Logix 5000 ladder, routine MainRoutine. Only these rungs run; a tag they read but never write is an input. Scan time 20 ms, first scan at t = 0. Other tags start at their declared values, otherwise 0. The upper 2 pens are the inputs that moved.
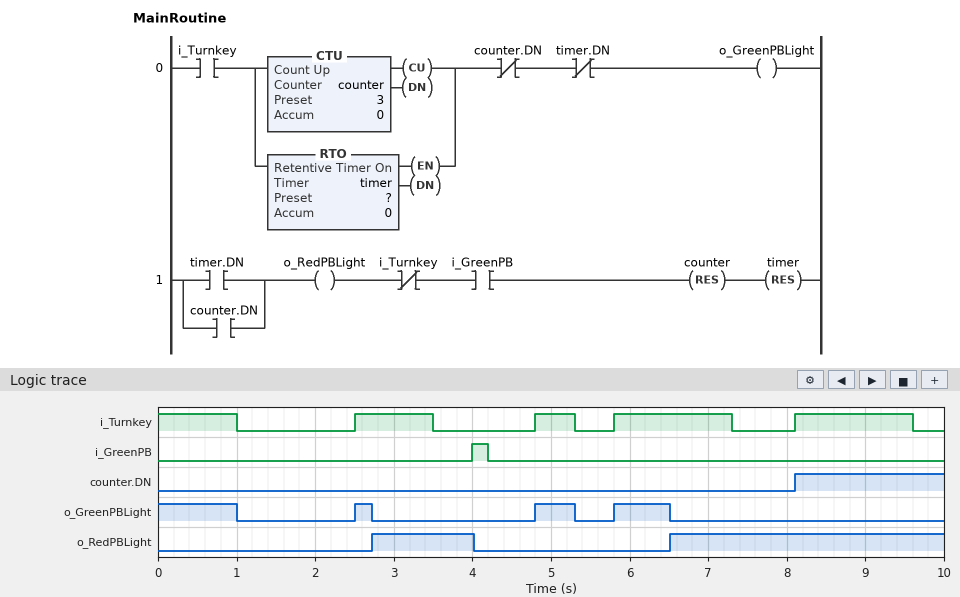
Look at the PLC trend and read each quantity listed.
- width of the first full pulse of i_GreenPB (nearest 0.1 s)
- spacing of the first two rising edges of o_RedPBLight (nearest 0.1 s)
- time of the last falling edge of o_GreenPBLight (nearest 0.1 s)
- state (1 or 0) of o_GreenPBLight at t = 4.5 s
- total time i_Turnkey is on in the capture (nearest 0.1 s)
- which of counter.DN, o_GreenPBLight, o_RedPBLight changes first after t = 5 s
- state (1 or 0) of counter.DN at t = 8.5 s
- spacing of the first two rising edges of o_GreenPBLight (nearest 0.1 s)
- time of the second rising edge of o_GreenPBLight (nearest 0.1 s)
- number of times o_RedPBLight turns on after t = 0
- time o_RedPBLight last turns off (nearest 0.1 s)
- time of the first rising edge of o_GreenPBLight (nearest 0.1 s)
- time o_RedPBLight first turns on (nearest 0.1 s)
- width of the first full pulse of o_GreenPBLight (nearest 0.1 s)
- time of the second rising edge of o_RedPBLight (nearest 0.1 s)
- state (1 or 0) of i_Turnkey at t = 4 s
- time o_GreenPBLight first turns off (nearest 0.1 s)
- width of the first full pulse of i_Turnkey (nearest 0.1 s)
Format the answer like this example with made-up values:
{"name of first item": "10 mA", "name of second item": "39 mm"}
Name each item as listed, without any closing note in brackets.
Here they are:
{"width of the first full pulse of i_GreenPB": "0.2 s", "spacing of the first two rising edges of o_RedPBLight": "3.8 s", "time of the last falling edge of o_GreenPBLight": "6.5 s", "state (1 or 0) of o_GreenPBLight at t = 4.5 s": "0", "total time i_Turnkey is on in the capture": "5.5 s", "which of counter.DN, o_GreenPBLight, o_RedPBLight changes first after t = 5 s": "o_GreenPBLight", "state (1 or 0) of counter.DN at t = 8.5 s": "1", "spacing of the first two rising edges of o_GreenPBLight": "2.3 s", "time of the second rising edge of o_GreenPBLight": "4.8 s", "number of times o_RedPBLight turns on after t = 0": "2", "time o_RedPBLight last turns off": "4.0 s", "time of the first rising edge of o_GreenPBLight": "2.5 s", "time o_RedPBLight first turns on": "2.7 s", "width of the first full pulse of o_GreenPBLight": "0.2 s", "time of the second rising edge of o_RedPBLight": "6.5 s", "state (1 or 0) of i_Turnkey at t = 4 s": "0", "time o_GreenPBLight first turns off": "1.0 s", "width of the first full pulse of i_Turnkey": "1.0 s"}
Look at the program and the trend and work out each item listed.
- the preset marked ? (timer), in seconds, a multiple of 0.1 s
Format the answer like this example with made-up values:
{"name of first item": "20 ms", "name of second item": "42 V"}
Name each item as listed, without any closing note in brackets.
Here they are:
{"the preset marked ? (timer), in seconds, a multiple of 0.1 s": "1.2 s"}
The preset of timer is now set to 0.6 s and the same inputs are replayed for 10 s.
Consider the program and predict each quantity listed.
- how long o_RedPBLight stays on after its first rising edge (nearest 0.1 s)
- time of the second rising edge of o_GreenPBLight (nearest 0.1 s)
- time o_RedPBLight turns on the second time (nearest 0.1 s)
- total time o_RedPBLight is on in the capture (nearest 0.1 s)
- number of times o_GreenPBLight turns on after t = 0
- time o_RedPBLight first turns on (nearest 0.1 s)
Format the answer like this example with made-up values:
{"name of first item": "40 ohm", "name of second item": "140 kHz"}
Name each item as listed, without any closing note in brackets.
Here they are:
{"how long o_RedPBLight stays on after its first rising edge": "3.4 s", "time of the second rising edge of o_GreenPBLight": "5.8 s", "time o_RedPBLight turns on the second time": "5.9 s", "total time o_RedPBLight is on in the capture": "7.5 s", "number of times o_GreenPBLight turns on after t = 0": "2", "time o_RedPBLight first turns on": "0.6 s"}
